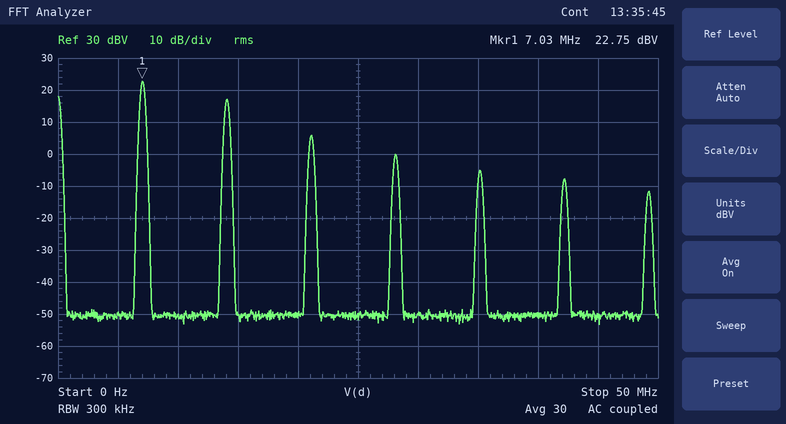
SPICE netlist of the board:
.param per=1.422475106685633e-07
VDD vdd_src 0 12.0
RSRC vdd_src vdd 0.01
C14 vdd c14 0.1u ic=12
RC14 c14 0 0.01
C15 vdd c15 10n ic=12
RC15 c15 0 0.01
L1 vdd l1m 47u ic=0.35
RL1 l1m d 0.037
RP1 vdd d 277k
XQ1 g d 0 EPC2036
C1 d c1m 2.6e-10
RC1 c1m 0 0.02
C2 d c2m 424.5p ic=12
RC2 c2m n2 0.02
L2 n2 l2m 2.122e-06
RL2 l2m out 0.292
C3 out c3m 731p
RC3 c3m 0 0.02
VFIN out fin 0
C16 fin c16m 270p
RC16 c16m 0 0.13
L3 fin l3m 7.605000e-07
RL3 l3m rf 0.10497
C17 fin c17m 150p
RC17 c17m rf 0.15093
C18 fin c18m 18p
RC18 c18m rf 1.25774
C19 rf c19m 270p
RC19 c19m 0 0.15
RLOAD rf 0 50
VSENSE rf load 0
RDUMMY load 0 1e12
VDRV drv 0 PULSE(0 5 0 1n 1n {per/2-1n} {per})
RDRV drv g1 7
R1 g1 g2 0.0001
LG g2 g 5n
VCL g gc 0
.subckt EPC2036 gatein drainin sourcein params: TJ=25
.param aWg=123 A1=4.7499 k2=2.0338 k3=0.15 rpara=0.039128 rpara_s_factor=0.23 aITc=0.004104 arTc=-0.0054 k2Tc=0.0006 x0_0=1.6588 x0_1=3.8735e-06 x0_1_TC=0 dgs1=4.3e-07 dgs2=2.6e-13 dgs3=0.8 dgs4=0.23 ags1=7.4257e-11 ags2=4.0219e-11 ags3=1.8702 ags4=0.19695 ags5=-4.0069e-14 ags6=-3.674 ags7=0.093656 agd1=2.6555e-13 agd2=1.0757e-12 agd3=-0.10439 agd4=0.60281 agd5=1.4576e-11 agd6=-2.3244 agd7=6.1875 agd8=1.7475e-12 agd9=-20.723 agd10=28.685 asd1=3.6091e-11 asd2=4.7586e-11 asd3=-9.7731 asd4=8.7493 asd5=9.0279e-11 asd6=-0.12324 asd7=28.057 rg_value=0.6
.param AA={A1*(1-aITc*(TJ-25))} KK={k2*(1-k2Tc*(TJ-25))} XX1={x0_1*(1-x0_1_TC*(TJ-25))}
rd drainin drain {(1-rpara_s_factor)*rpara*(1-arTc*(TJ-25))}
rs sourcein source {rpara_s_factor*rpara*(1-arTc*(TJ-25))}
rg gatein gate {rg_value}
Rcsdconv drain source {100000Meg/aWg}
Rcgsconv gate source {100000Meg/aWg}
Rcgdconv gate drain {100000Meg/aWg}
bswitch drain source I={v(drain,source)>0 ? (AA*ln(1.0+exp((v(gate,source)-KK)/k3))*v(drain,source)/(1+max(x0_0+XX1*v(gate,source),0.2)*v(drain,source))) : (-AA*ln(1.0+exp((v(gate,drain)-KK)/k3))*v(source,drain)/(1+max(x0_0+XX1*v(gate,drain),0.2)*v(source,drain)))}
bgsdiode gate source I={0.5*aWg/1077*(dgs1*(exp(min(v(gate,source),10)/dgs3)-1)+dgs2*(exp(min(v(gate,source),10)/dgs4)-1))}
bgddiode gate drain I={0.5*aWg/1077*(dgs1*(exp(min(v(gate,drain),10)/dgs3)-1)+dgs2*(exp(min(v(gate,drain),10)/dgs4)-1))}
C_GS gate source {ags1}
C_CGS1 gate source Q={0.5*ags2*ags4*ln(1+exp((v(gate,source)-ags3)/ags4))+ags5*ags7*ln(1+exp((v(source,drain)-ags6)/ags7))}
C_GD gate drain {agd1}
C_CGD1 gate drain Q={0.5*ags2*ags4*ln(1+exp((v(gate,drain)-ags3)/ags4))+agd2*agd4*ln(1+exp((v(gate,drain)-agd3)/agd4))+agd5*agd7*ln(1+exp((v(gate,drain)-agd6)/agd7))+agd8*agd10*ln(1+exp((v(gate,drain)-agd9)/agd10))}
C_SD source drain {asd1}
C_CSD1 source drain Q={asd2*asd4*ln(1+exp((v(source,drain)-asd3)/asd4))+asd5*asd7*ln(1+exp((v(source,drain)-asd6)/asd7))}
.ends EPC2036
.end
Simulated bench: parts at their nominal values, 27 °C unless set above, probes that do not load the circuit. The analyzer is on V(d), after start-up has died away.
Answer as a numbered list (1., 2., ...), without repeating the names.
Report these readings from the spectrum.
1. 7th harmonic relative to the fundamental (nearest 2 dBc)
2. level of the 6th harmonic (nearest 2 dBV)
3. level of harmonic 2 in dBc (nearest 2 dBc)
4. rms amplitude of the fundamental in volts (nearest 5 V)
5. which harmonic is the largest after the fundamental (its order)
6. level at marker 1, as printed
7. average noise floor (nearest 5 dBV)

1. -34 dBc
2. -8 dBV
3. -6 dBc
4. 15 V
5. 2
6. 22.75 dBV
7. -50 dBV
